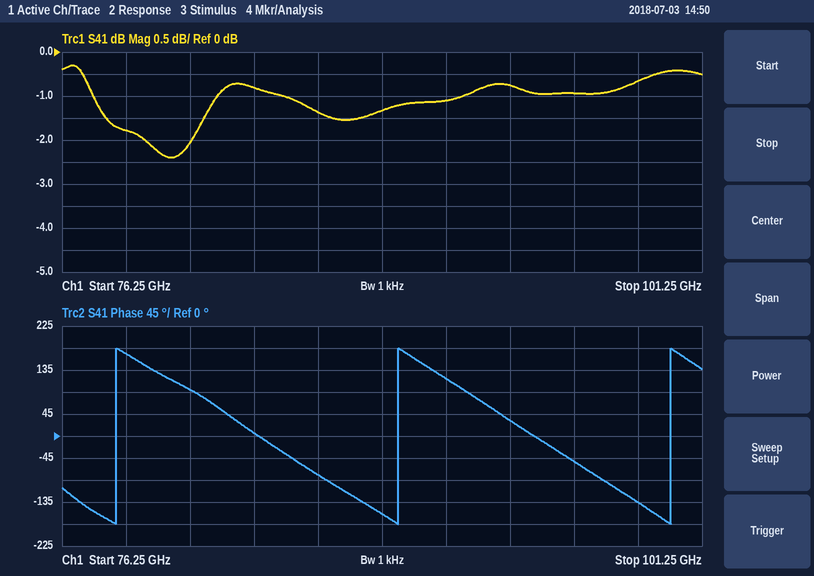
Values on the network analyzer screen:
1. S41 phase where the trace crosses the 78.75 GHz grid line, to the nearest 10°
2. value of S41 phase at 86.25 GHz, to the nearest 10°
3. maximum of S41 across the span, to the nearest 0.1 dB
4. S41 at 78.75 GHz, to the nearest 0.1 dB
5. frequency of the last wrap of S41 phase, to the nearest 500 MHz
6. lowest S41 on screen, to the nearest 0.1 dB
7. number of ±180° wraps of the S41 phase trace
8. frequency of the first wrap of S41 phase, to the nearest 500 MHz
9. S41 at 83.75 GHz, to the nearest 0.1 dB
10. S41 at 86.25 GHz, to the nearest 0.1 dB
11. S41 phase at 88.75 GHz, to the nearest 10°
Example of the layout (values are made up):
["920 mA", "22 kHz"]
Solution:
["170°", "-80°", "-0.3 dB", "-1.8 dB", "100.0 GHz", "-2.4 dB", "3", "78.5 GHz", "-0.8 dB", "-1.4 dB", "-160°"]
